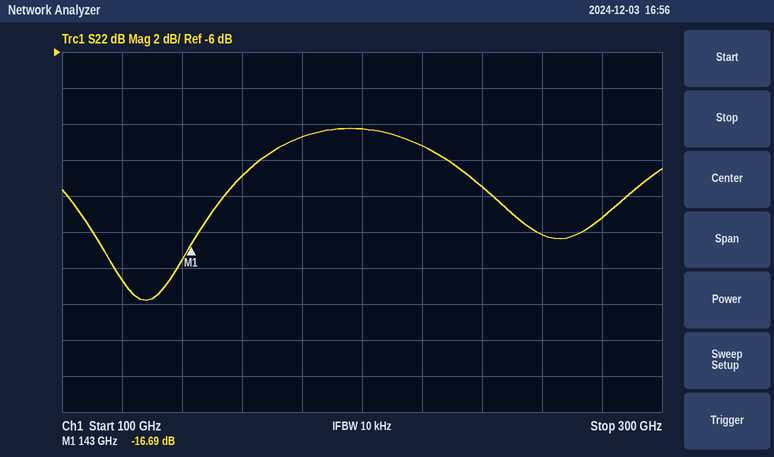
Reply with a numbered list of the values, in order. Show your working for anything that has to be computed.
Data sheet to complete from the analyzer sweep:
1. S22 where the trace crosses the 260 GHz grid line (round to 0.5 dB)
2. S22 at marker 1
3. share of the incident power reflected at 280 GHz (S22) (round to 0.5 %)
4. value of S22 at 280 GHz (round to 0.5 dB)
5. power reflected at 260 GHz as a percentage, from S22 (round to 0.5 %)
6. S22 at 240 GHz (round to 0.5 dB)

1. -16.0 dB
2. -16.69 dB
3. 10^(-15/10) ≈ 3.16 %, so 3.0 % to the nearest 0.5 %
4. -15.0 dB
5. 10^(-16/10) ≈ 2.5 %
6. -13.5 dB
